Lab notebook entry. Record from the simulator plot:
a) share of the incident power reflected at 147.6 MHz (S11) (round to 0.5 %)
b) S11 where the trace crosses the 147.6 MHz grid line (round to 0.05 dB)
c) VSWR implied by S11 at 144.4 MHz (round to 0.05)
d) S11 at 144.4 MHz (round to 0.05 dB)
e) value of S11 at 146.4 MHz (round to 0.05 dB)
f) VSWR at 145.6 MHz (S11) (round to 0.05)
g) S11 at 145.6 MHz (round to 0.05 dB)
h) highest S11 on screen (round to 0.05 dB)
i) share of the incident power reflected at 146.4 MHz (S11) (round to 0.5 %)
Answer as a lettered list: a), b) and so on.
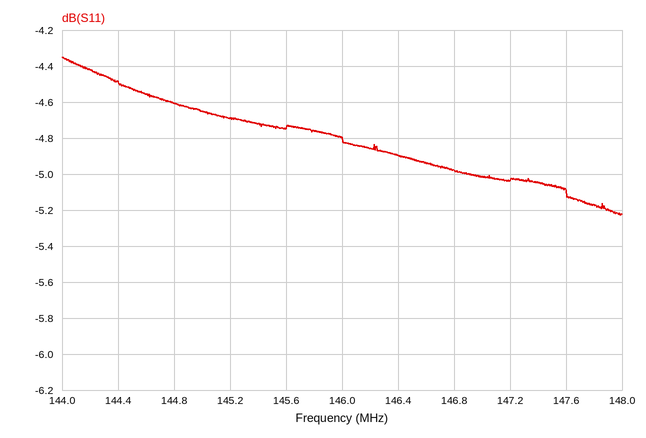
a) 31.0 %
b) -5.10 dB
c) 3.95
d) -4.50 dB
e) -4.90 dB
f) 3.75
g) -4.75 dB
h) -4.35 dB
i) 32.5 %
